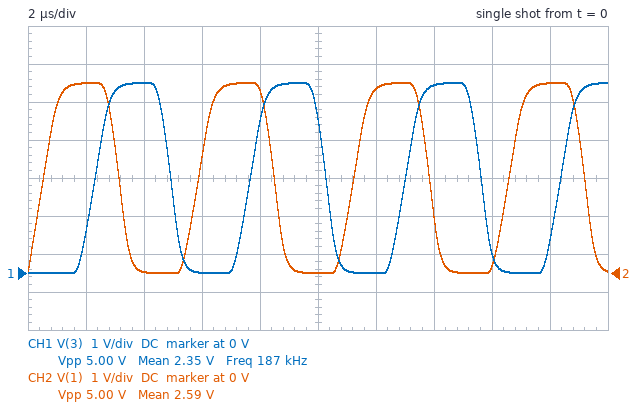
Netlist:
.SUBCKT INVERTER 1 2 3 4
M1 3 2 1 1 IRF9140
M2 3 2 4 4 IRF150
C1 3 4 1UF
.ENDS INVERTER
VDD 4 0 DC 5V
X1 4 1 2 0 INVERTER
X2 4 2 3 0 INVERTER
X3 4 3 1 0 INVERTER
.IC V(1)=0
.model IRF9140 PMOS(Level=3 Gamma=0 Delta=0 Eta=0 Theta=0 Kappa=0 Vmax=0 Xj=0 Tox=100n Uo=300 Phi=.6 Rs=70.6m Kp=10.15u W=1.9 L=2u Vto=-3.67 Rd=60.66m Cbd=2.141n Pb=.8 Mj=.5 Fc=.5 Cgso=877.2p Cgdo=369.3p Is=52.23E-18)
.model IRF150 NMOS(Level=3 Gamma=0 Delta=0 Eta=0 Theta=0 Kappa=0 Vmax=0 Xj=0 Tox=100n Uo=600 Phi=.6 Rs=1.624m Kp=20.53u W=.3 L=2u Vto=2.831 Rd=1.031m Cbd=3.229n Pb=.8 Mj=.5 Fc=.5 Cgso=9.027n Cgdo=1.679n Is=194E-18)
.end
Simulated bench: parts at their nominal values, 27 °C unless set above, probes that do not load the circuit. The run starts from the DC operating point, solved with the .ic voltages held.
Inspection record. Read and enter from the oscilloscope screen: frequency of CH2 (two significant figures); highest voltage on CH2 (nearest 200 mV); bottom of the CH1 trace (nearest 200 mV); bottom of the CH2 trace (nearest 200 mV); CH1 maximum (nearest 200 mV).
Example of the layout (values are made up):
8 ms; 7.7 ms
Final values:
190 kHz; 5.0 V; 0 V; 0 V; 5.0 V
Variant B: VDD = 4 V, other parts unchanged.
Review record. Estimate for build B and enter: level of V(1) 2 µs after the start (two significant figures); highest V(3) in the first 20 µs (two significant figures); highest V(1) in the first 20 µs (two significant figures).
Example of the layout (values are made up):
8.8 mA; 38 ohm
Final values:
850 mV; 3.9 V; 4.0 V
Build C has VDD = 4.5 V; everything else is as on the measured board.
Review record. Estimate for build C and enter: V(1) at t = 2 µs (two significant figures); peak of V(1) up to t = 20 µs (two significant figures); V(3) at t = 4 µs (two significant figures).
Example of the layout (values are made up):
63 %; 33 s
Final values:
4.2 V; 4.5 V; 1.9 V
